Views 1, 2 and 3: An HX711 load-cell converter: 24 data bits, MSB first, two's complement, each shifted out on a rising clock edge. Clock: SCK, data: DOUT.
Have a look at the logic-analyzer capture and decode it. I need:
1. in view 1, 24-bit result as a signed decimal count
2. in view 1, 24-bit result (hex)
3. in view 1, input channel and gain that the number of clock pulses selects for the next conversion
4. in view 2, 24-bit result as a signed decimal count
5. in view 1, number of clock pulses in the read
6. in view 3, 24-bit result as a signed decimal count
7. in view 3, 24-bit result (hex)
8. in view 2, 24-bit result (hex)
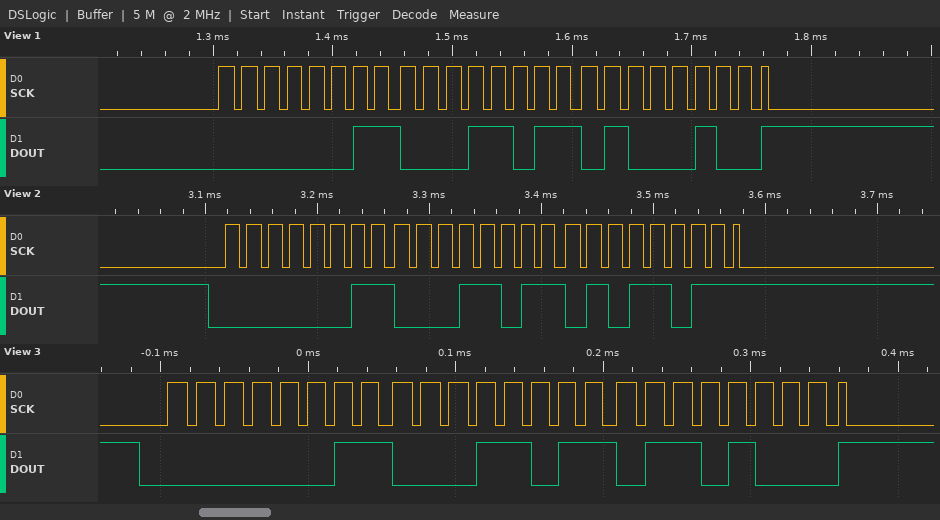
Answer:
203588
0x031B44
channel A, gain 128
203611
25
203624
0x031B68
0x031B5B
